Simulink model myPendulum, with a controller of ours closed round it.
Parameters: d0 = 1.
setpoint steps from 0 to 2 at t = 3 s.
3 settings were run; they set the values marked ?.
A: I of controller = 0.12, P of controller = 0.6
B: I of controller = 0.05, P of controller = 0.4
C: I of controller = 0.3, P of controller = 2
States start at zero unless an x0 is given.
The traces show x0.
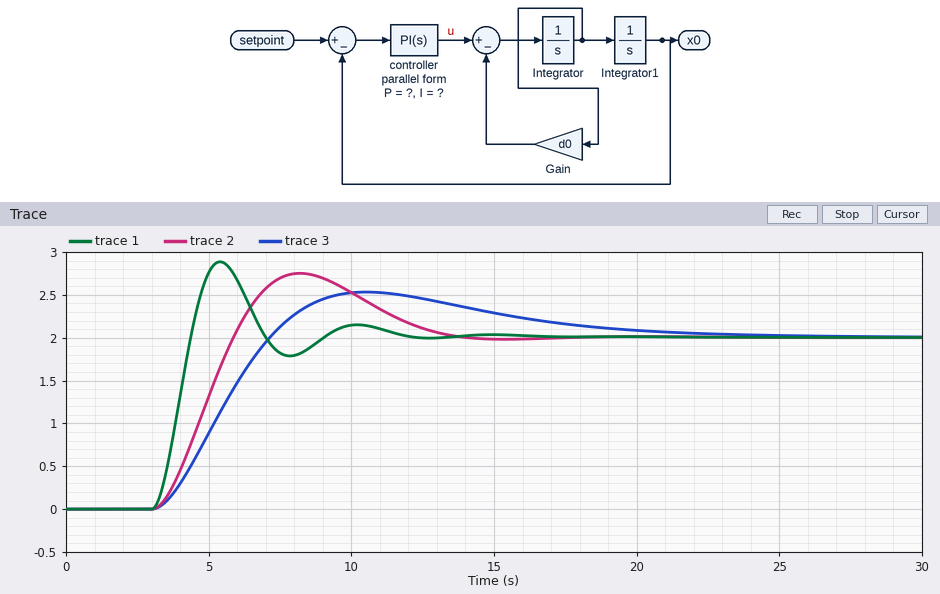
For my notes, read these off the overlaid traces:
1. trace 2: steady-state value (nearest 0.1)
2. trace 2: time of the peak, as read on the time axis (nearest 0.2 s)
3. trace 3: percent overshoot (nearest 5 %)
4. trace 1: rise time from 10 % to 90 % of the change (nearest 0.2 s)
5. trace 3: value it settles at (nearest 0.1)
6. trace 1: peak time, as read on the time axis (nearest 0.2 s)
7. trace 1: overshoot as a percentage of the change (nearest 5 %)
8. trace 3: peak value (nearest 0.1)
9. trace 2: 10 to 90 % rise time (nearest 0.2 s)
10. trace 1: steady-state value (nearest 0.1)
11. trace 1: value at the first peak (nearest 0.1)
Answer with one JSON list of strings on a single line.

["2.0", "8.2 s", "25 %", "1.0 s", "2.0", "5.4 s", "45 %", "2.5", "2.0 s", "2.0", "2.9"]
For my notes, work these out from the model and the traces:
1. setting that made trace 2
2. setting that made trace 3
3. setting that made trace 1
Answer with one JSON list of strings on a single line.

["A", "B", "C"]
